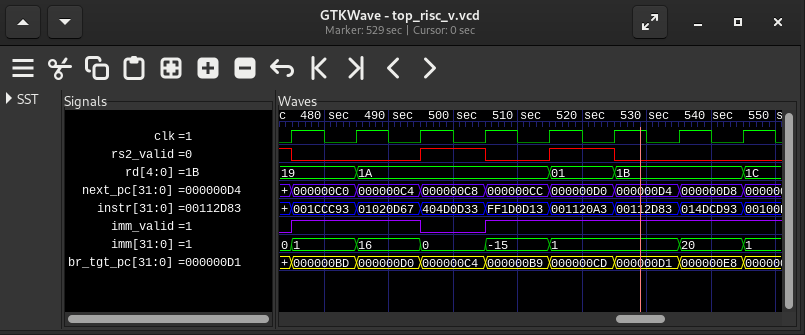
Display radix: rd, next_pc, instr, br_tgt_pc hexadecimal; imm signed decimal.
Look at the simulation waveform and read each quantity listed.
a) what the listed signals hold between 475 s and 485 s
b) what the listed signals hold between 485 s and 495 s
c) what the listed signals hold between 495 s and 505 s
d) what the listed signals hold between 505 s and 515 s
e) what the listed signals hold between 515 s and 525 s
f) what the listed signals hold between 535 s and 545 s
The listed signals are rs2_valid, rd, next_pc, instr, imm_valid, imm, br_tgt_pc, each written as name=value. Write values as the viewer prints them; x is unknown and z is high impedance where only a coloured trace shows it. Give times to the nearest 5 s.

rs2_valid=0, rd=19, next_pc=000000C0, instr=001CCC93, imm_valid=1, imm=1, br_tgt_pc=000000BD
rs2_valid=0, rd=1A, next_pc=000000C4, instr=01020D67, imm_valid=1, imm=16, br_tgt_pc=000000D0
rs2_valid=1, rd=1A, next_pc=000000C8, instr=404D0D33, imm_valid=0, imm=0, br_tgt_pc=000000C4
rs2_valid=0, rd=1A, next_pc=000000CC, instr=FF1D0D13, imm_valid=1, imm=-15, br_tgt_pc=000000B9
rs2_valid=1, rd=01, next_pc=000000D0, instr=001120A3, imm_valid=1, imm=1, br_tgt_pc=000000CD
rs2_valid=0, rd=1B, next_pc=000000D8, instr=014DCD93, imm_valid=1, imm=20, br_tgt_pc=000000E8
